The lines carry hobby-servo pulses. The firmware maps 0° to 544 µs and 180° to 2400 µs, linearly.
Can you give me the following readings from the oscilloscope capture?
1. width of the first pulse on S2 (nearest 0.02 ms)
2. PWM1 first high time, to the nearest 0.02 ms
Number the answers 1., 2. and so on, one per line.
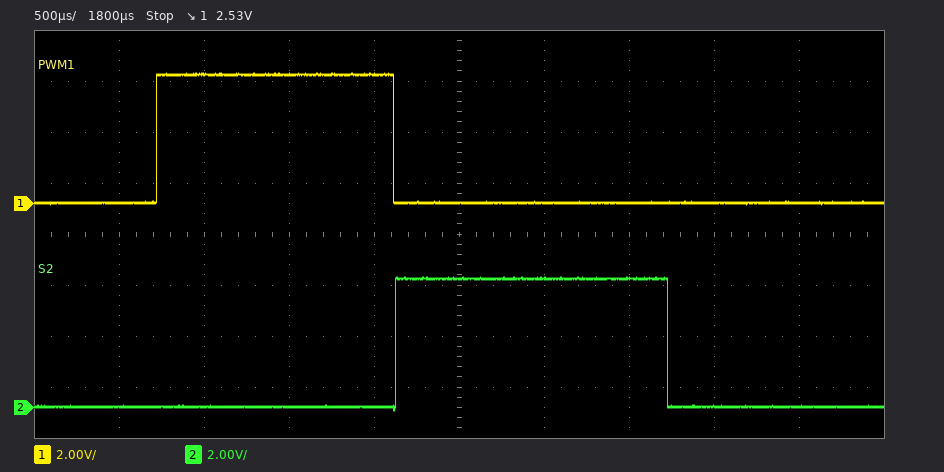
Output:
1. 1.60 ms
2. 1.40 ms
